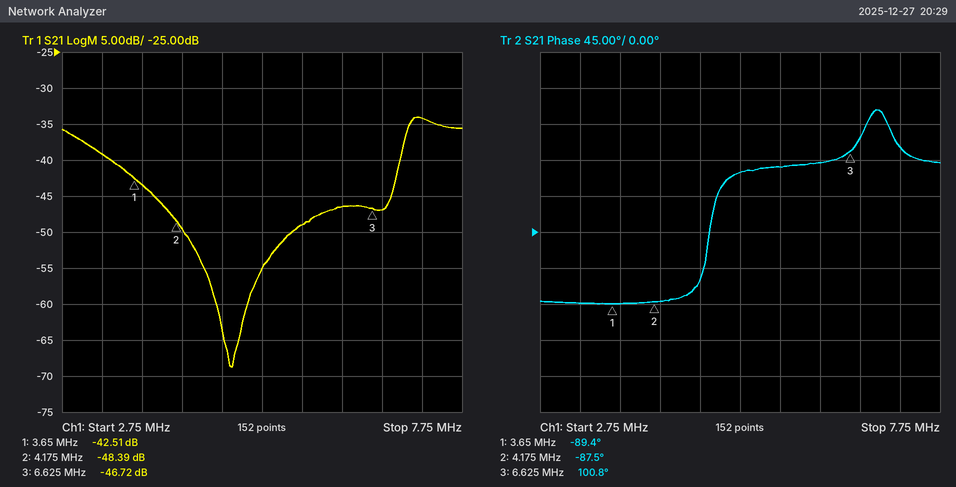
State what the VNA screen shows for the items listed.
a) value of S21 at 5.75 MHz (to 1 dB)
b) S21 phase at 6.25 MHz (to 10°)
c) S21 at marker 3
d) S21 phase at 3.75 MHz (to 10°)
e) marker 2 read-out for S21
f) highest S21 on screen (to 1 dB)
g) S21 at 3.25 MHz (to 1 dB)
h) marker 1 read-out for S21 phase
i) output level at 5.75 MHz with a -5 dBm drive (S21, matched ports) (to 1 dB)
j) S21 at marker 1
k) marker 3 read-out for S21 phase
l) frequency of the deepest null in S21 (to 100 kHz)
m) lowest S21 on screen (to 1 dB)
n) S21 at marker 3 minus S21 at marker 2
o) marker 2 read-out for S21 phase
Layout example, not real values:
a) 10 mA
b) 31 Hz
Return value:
a) -49 dB
b) 90°
c) -46.72 dB
d) -90°
e) -48.39 dB
f) -34 dB
g) -39 dB
h) -89.4°
i) -54 dBm
j) -42.51 dB
k) 100.8°
l) 4.9 MHz
m) -69 dB
n) 1.67 dB
o) -87.5°
